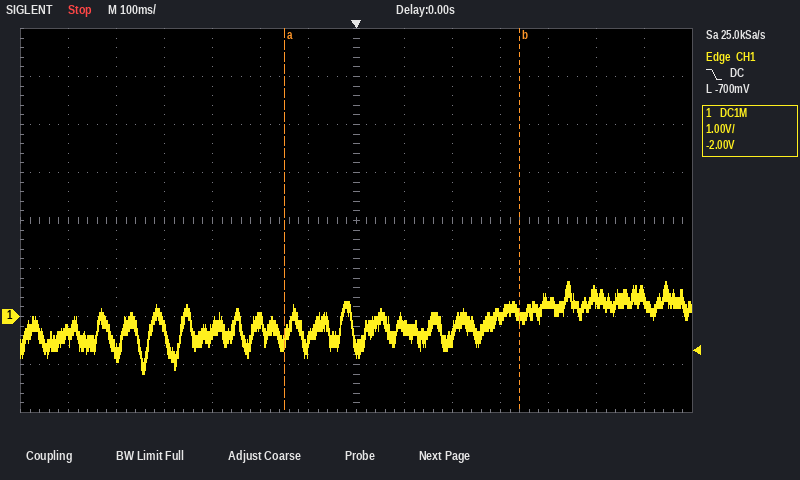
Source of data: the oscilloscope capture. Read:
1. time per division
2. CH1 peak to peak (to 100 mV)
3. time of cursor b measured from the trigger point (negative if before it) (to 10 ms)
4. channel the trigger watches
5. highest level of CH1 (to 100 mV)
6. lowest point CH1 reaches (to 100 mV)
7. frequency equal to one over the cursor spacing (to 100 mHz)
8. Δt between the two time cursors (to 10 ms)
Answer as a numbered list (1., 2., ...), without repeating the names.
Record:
1. 100 ms
2. 1.9 V
3. +340 ms
4. CH1
5. 700 mV
6. -1.2 V
7. 2.0 Hz
8. 490 ms
